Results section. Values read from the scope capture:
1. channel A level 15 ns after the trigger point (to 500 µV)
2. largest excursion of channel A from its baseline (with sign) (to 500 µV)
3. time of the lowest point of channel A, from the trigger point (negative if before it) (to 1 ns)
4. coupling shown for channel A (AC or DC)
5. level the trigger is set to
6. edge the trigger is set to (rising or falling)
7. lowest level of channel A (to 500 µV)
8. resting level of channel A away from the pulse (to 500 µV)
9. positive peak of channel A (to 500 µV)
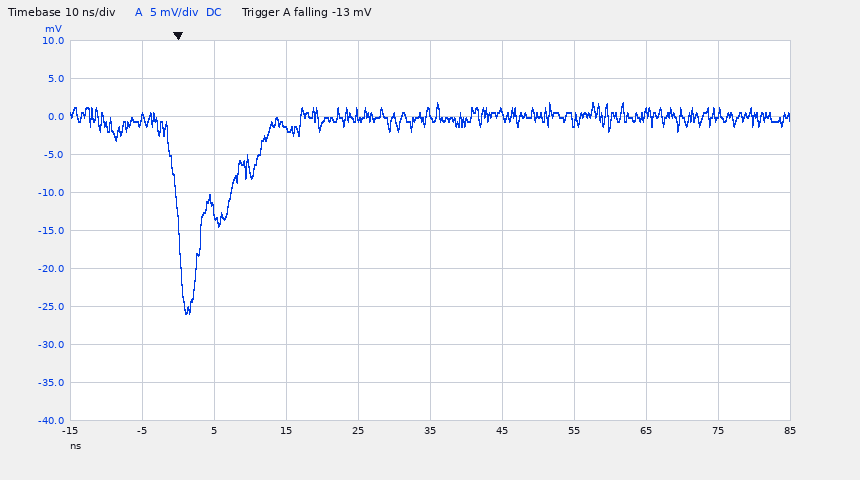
-1.5 mV
-26.0 mV
+1 ns
DC
-13 mV
falling
-26.0 mV
0.0 mV
2.0 mV
